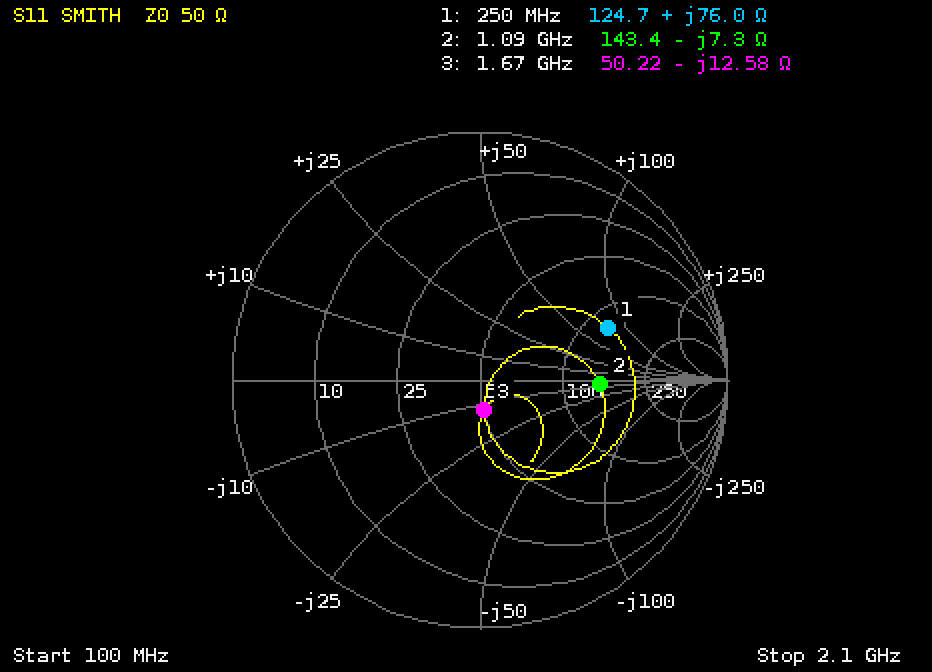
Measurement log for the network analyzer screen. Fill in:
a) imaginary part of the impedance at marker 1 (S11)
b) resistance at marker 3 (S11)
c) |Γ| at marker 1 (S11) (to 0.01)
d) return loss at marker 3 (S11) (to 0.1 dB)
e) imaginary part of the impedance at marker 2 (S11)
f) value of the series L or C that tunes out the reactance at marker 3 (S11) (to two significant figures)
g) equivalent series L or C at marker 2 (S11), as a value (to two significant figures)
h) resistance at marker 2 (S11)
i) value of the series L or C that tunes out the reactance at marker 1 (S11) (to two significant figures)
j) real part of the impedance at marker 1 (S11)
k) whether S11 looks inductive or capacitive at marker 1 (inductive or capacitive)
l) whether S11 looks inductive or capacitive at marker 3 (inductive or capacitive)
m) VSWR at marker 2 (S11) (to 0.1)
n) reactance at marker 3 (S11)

+76.0 Ω
50.22 Ω
0.56
18.1 dB
-7.3 Ω
1.2 nH
20 pF
143.4 Ω
8.4 pF
124.7 Ω
inductive
capacitive
2.9
-12.58 Ω
